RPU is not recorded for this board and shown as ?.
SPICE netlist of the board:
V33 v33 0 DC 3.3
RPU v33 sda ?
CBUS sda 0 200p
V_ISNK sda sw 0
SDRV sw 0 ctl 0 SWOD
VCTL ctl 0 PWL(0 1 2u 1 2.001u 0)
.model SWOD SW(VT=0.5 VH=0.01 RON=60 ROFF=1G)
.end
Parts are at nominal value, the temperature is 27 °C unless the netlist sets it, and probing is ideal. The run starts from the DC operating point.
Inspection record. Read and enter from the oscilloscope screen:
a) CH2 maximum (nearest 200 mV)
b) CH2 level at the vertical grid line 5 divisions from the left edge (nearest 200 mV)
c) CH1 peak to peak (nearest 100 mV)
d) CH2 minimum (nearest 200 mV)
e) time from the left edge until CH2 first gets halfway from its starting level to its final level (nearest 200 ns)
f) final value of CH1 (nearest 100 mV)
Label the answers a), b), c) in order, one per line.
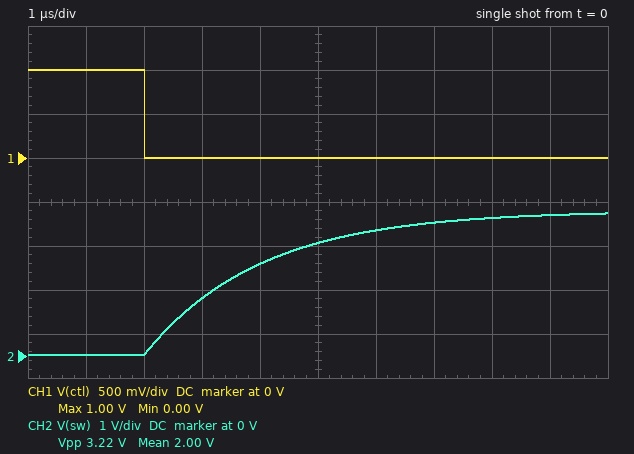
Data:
a) 3.2 V
b) 2.6 V
c) 1.0 V
d) 0 V
e) 3.4 µs
f) 0 V
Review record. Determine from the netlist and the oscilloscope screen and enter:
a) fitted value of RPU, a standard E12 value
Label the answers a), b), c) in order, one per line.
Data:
a) 10 kΩ
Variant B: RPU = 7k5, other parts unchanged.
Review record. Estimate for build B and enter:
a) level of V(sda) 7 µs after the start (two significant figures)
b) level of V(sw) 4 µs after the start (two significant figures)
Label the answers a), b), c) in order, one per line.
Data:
a) 3.2 V
b) 2.4 V
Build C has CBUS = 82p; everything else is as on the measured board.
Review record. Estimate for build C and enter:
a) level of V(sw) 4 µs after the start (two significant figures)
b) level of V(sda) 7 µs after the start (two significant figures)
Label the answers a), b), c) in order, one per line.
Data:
a) 3.0 V
b) 3.3 V
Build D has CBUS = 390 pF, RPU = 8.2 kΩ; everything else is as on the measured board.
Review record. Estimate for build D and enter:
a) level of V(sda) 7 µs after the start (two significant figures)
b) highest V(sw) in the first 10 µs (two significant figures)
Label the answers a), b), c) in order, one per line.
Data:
a) 2.6 V
b) 3.0 V
